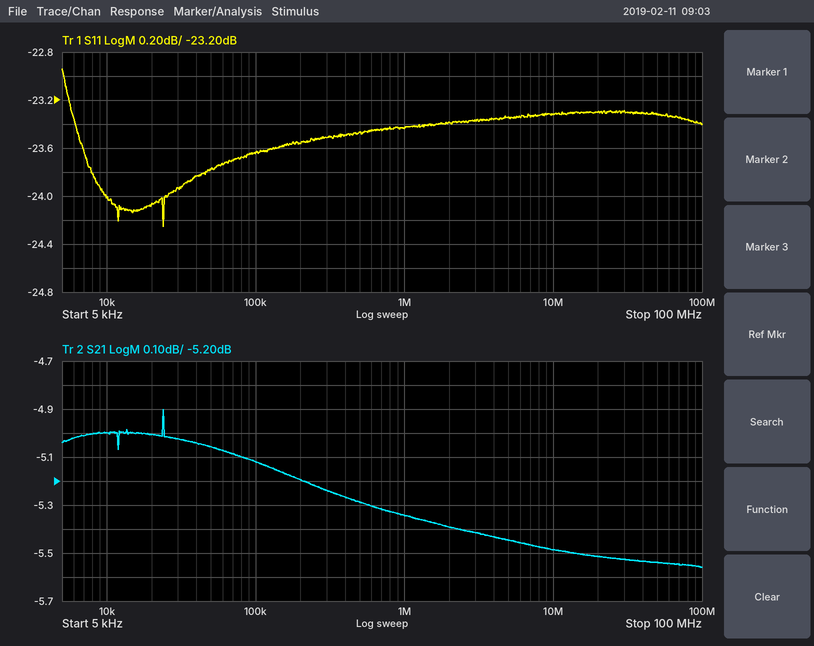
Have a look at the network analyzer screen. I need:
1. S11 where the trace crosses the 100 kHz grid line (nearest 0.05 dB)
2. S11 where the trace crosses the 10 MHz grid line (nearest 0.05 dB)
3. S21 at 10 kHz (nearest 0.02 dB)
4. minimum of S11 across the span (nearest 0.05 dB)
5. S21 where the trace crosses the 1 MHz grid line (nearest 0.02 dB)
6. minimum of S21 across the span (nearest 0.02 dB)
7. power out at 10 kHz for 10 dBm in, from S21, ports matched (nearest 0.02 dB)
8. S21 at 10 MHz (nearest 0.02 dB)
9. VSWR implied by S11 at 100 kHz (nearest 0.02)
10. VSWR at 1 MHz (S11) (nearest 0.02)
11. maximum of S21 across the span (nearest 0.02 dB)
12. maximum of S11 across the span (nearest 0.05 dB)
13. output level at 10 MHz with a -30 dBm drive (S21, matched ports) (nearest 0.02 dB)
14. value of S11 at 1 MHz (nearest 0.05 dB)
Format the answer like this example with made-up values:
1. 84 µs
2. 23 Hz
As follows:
1. -23.65 dB
2. -23.30 dB
3. -5.00 dB
4. -24.25 dB
5. -5.34 dB
6. -5.56 dB
7. 5.00 dBm
8. -5.48 dB
9. 1.14
10. 1.14
11. -4.90 dB
12. -22.95 dB
13. -35.48 dBm
14. -23.45 dB
